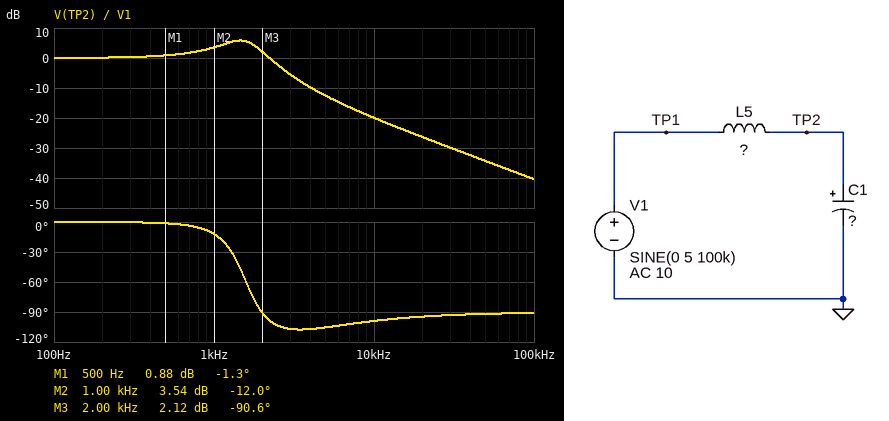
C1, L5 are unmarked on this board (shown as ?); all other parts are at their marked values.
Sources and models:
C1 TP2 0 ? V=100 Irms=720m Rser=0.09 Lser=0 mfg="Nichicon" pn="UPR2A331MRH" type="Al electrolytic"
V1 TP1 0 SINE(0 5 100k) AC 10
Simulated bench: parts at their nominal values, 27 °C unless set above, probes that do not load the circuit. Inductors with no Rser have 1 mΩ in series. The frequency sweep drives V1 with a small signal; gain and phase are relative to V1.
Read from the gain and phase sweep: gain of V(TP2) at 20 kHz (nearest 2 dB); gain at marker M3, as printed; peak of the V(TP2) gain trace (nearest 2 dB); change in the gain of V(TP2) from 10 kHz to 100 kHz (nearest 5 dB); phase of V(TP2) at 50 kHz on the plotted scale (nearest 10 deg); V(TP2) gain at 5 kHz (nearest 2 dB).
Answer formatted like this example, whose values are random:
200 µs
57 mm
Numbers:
-26 dB
2.12 dB
6 dB
-20 dB
-90 deg
-12 dB
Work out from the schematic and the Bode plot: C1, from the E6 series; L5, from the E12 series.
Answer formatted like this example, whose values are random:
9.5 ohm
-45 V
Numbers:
680 µF
15 µH
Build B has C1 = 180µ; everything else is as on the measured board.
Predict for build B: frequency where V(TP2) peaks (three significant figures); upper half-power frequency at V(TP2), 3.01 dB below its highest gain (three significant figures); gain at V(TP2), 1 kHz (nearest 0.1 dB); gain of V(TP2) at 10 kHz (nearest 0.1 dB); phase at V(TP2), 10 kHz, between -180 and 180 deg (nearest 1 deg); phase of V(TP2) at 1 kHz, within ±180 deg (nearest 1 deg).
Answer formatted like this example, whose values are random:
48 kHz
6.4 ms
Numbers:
2.99 kHz
3.45 kHz
1.0 dB
-16.7 dB
-128 deg
-1 deg
